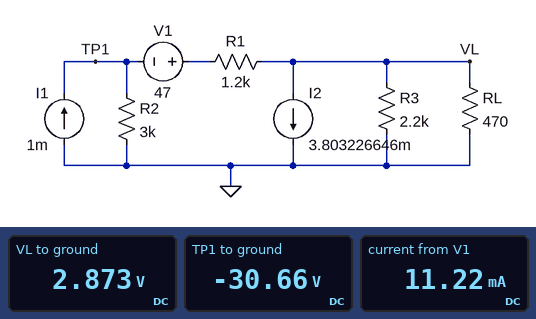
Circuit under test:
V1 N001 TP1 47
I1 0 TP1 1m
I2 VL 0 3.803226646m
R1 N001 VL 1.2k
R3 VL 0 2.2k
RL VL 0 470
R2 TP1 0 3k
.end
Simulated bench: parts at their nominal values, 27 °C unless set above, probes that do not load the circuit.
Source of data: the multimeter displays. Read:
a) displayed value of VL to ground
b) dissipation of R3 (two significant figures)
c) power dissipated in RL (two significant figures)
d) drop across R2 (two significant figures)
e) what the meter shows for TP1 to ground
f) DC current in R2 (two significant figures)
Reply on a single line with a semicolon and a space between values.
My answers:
2.873 V; 3.8 mW; 18 mW; 31 V; -30.66 V; 10 mA
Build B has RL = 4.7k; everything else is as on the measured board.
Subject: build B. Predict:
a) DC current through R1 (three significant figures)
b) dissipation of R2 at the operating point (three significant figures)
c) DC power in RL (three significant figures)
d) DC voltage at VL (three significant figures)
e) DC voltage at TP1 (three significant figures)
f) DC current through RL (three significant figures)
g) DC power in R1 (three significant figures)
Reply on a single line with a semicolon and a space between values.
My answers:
9.77 mA; 231 mW; 17.0 mW; 8.95 V; -26.3 V; 1.90 mA; 115 mW
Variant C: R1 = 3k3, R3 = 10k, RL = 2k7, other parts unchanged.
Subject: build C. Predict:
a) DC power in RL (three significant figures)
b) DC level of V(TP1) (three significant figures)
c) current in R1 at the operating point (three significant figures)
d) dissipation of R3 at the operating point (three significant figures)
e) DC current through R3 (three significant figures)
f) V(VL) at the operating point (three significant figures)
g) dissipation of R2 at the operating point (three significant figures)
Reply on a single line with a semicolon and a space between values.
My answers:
16.0 mW; -17.7 V; 6.89 mA; 4.32 mW; 657 µA; 6.57 V; 104 mW
